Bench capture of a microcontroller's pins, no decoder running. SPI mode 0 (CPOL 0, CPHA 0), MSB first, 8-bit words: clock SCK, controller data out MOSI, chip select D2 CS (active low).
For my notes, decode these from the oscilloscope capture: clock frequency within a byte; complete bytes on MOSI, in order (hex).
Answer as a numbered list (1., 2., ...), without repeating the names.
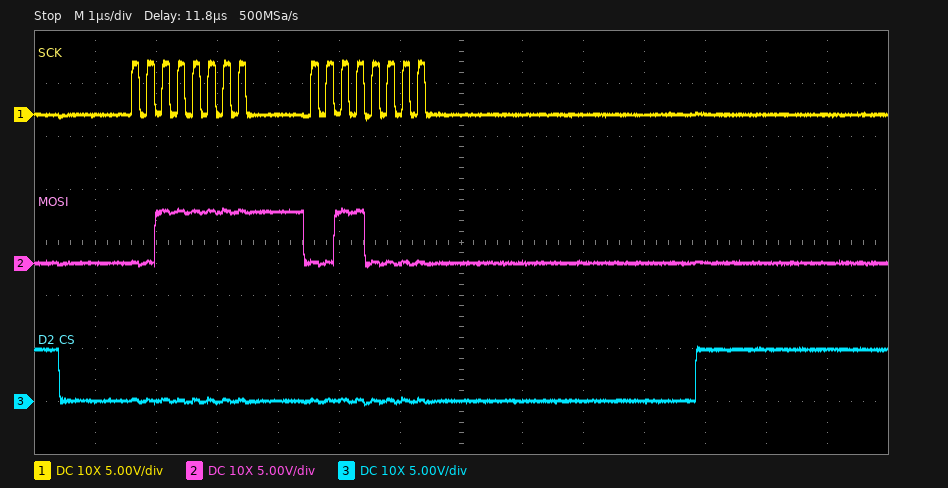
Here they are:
1. 4 MHz
2. 3F 30
